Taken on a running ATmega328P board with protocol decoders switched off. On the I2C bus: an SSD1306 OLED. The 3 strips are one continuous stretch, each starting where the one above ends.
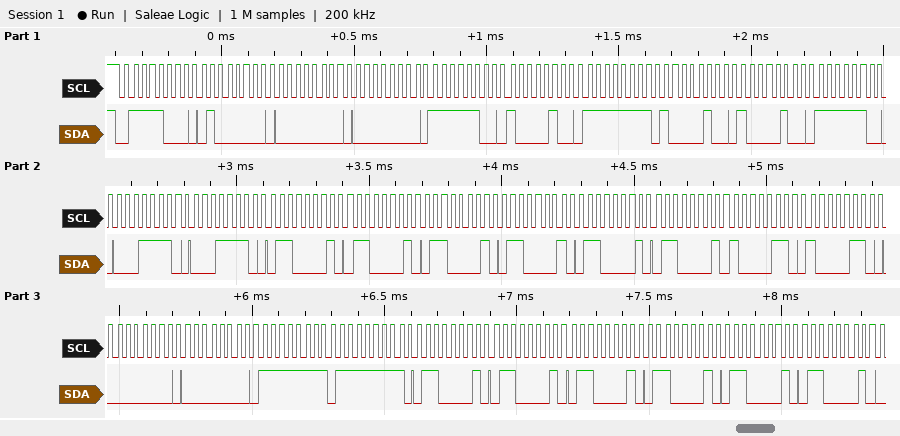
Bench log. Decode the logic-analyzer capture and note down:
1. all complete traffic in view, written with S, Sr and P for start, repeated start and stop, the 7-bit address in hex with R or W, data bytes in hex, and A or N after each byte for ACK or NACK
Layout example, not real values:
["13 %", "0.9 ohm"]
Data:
["S 3CW A 40 A 00 A 00 A FC A 84 A FF A 84 A 84 A FC A 1E A 1E A 61 A 61 A 61 A 61 A 61 A 61 A 86 A 86 A 00 A 00 A FF A FF A 61 A 61 A 61 A 61 A 61 A 61 A"]
